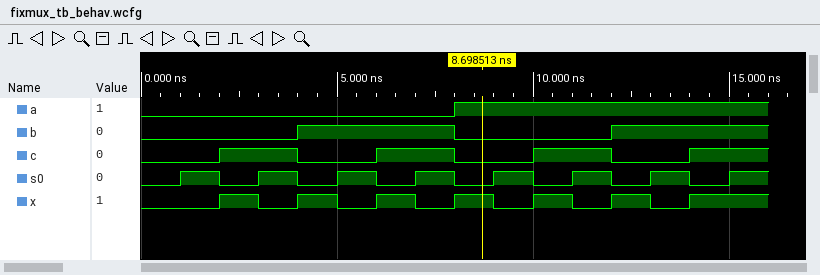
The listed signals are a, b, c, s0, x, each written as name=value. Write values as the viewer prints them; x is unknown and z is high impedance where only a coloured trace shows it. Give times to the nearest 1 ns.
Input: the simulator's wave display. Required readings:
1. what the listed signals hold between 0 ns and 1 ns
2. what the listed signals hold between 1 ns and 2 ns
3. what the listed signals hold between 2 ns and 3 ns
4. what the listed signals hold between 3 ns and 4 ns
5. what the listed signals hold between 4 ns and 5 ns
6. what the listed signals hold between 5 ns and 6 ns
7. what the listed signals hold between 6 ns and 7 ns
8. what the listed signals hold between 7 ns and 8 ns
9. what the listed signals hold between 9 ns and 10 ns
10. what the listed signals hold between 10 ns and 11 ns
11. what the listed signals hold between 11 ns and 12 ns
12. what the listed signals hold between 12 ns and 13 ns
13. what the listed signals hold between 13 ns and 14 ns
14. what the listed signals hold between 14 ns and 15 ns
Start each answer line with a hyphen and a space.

- a=0, b=0, c=0, s0=0, x=0
- a=0, b=0, c=0, s0=1, x=0
- a=0, b=0, c=1, s0=0, x=1
- a=0, b=0, c=1, s0=1, x=0
- a=0, b=1, c=0, s0=0, x=1
- a=0, b=1, c=0, s0=1, x=0
- a=0, b=1, c=1, s0=0, x=1
- a=0, b=1, c=1, s0=1, x=0
- a=1, b=0, c=0, s0=1, x=0
- a=1, b=0, c=1, s0=0, x=1
- a=1, b=0, c=1, s0=1, x=0
- a=1, b=1, c=0, s0=0, x=1
- a=1, b=1, c=0, s0=1, x=0
- a=1, b=1, c=1, s0=0, x=1
